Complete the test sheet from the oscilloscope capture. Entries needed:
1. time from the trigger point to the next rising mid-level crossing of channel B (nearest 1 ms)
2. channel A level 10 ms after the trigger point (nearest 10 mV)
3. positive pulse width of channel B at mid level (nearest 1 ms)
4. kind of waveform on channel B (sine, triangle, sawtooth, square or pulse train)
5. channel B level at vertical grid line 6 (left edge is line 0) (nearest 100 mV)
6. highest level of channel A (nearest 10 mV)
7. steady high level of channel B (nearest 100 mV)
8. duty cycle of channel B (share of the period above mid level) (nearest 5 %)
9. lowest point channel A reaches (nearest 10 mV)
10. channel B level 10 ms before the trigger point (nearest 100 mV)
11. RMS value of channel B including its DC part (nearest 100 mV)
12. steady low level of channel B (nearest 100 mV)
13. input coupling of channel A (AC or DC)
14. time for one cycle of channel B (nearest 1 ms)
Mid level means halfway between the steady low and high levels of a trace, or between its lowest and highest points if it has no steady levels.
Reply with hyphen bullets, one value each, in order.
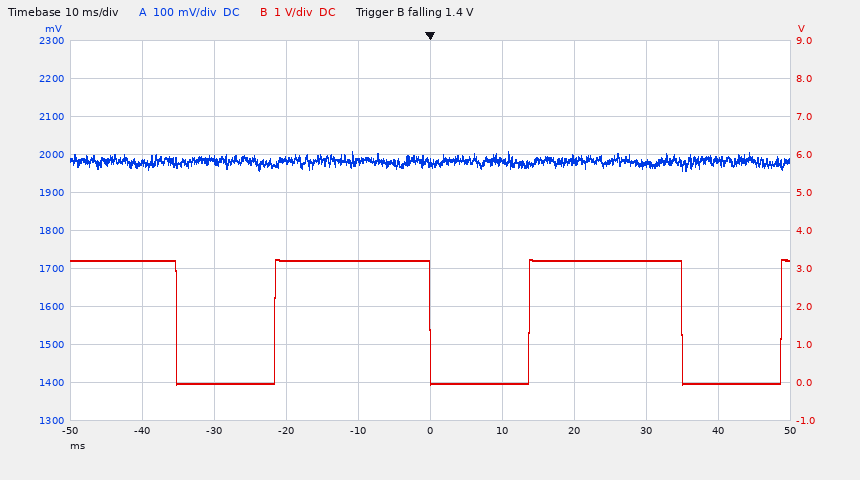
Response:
- 14 ms
- 1.98 V
- 21 ms
- pulse train
- 0.0 V
- 2.01 V
- 3.2 V
- 60 %
- 1.96 V
- 3.2 V
- 2.5 V
- 0.0 V
- DC
- 35 ms
